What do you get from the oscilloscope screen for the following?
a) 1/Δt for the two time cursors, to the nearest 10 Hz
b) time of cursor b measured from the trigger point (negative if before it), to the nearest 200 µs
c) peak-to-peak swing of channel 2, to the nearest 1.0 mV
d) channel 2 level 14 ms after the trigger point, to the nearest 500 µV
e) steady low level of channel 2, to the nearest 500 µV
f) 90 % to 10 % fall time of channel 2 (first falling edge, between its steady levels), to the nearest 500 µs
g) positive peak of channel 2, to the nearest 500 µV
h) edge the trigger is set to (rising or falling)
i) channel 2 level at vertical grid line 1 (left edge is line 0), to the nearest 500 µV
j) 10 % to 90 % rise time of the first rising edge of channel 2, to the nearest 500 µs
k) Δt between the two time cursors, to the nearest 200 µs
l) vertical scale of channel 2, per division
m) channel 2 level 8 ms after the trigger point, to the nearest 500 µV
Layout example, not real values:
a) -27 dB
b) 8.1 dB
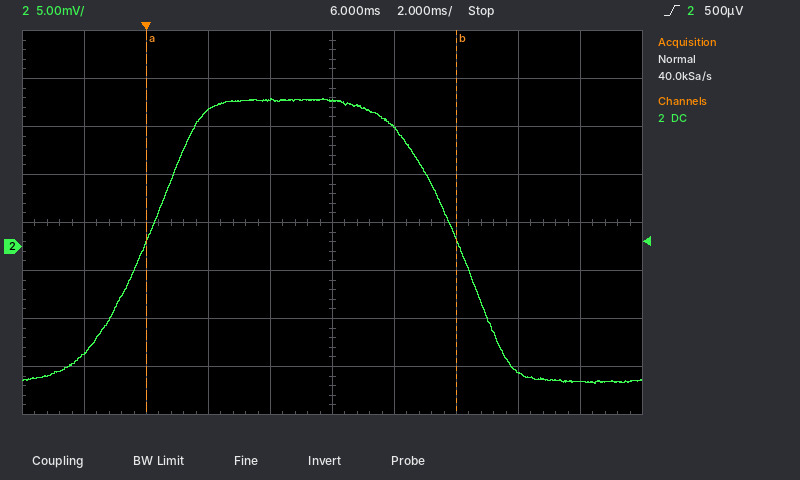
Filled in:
a) 100 Hz
b) +10.0 ms
c) 30.0 mV
d) -14.0 mV
e) -14.0 mV
f) 3.5 ms
g) 15.5 mV
h) rising
i) -11.0 mV
j) 3.5 ms
k) 10.0 ms
l) 5 mV
m) 12.5 mV
